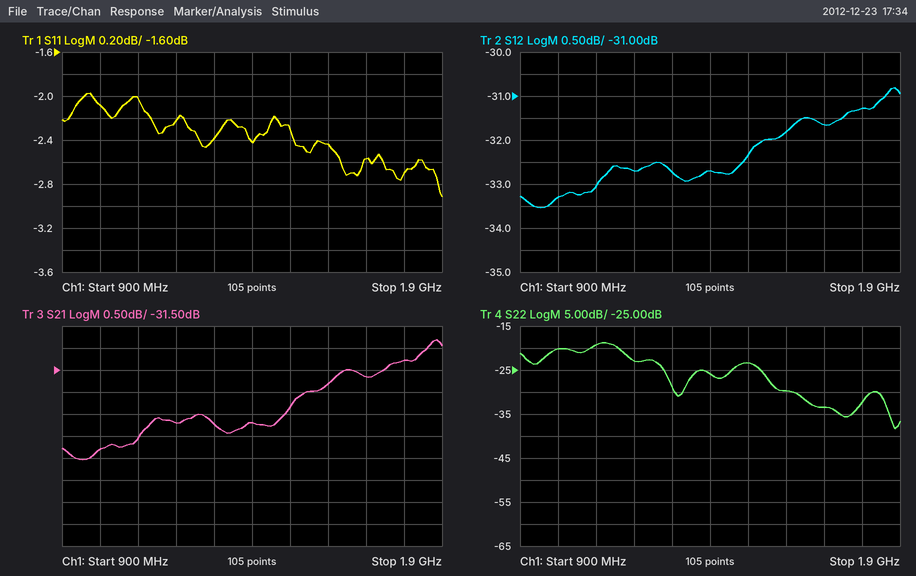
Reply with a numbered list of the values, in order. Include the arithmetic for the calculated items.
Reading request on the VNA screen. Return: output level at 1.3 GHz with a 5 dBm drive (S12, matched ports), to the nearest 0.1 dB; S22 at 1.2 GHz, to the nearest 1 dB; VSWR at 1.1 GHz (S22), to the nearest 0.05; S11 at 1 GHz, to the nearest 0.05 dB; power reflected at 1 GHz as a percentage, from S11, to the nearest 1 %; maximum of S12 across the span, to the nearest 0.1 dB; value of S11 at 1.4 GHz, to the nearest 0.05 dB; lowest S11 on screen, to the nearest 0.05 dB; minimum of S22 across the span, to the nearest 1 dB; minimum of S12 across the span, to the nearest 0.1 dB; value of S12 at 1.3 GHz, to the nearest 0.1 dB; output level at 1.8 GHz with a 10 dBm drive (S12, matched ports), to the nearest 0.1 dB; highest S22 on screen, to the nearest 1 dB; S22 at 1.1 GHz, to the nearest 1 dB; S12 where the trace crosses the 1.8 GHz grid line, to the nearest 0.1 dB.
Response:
1. 5 dBm + (-32.7 dB) = -27.7 dBm
2. -23 dB
3. |Γ| = 10^(-19/20) = 0.1122; VSWR = (1 + 0.1122)/(1 − 0.1122) ≈ 1.25
4. -2.10 dB
5. 10^(-2.1/10) ≈ 62 %
6. -30.8 dB
7. -2.40 dB
8. -2.90 dB
9. -38 dB
10. -33.5 dB
11. -32.7 dB
12. 10 dBm + (-31.3 dB) = -21.3 dBm
13. -19 dB
14. -19 dB
15. -31.3 dB
